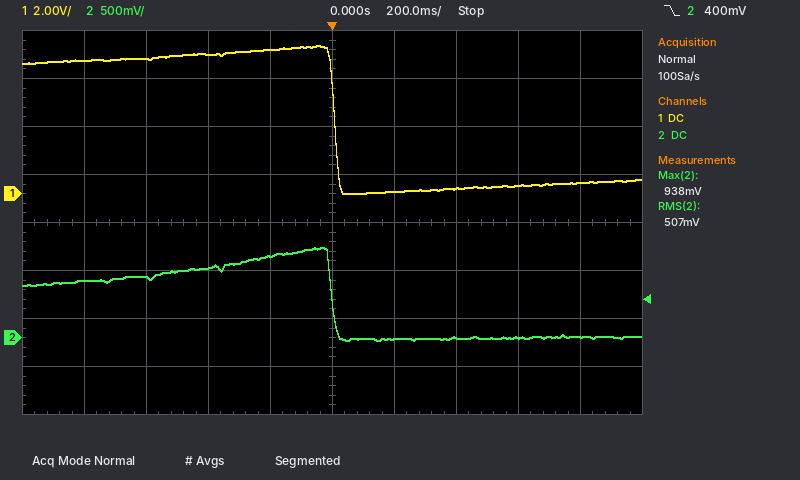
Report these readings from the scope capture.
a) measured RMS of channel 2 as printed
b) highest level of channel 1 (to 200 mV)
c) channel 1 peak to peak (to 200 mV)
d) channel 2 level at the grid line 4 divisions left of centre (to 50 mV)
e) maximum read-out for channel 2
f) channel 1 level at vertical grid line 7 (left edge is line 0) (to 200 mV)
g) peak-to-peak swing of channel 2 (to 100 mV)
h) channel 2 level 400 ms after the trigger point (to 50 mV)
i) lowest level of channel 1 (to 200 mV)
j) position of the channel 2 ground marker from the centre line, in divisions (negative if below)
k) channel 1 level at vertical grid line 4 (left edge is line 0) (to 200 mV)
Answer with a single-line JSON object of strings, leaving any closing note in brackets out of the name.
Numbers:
{"measured RMS of channel 2 as printed": "507 mV", "highest level of channel 1": "6.2 V", "channel 1 peak to peak": "6.2 V", "channel 2 level at the grid line 4 divisions left of centre": "600 mV", "maximum read-out for channel 2": "938 mV", "channel 1 level at vertical grid line 7 (left edge is line 0)": "200 mV", "peak-to-peak swing of channel 2": "1.00 V", "channel 2 level 400 ms after the trigger point": "0 mV", "lowest level of channel 1": "0.0 V", "position of the channel 2 ground marker from the centre line, in divisions": "-2.4 div", "channel 1 level at vertical grid line 4 (left edge is line 0)": "6.0 V"}
